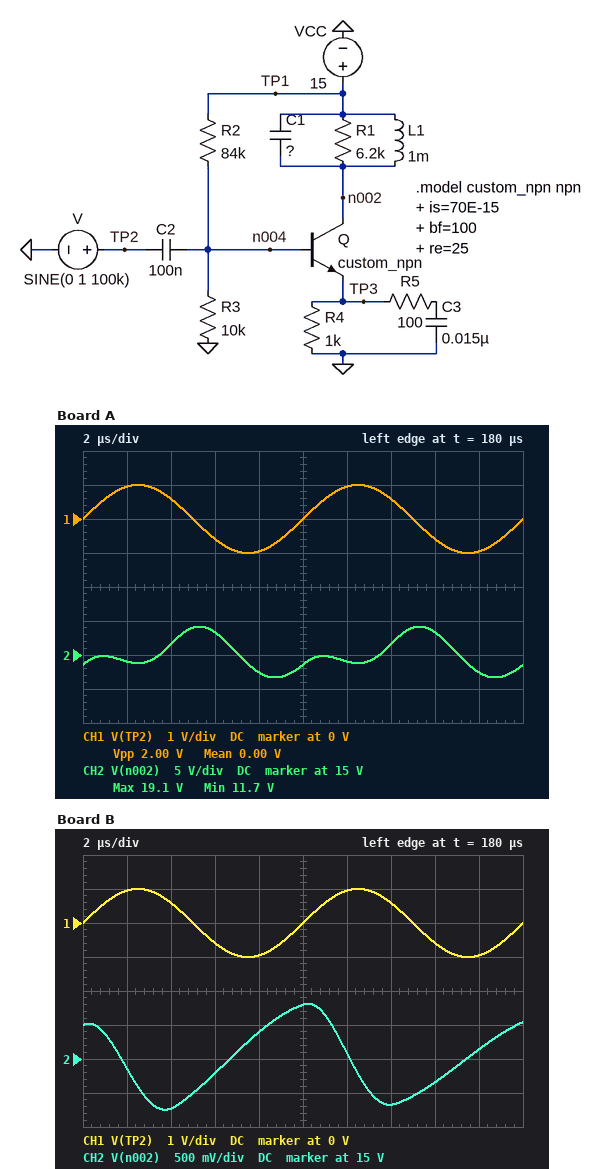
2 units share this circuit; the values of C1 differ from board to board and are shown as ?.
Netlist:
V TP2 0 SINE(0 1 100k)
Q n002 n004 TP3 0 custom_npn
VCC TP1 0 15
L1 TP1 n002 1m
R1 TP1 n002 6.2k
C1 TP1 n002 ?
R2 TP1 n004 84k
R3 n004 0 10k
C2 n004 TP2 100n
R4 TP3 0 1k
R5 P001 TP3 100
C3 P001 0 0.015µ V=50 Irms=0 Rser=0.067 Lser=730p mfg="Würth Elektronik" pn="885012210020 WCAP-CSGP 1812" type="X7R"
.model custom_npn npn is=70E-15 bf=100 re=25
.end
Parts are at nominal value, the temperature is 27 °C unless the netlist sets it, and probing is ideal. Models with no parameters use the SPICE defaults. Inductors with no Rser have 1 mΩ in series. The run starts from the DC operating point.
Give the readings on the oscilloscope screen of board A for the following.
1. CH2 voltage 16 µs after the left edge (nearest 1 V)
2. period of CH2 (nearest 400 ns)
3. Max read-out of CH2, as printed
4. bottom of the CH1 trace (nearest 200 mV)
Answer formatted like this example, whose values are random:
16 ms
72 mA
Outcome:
18 V
10.0 µs
19.1 V
-1.0 V
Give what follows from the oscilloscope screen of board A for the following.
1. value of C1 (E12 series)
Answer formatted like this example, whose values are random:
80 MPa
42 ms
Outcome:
1.2 nF
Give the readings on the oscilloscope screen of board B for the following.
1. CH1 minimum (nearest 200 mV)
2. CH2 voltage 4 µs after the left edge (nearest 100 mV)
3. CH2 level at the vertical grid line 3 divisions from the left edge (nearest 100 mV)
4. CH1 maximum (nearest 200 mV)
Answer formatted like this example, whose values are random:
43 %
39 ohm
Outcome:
-1.0 V
14.3 V
14.8 V
1.0 V
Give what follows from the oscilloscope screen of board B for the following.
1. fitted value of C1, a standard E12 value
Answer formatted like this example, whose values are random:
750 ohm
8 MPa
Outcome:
8.2 nF
